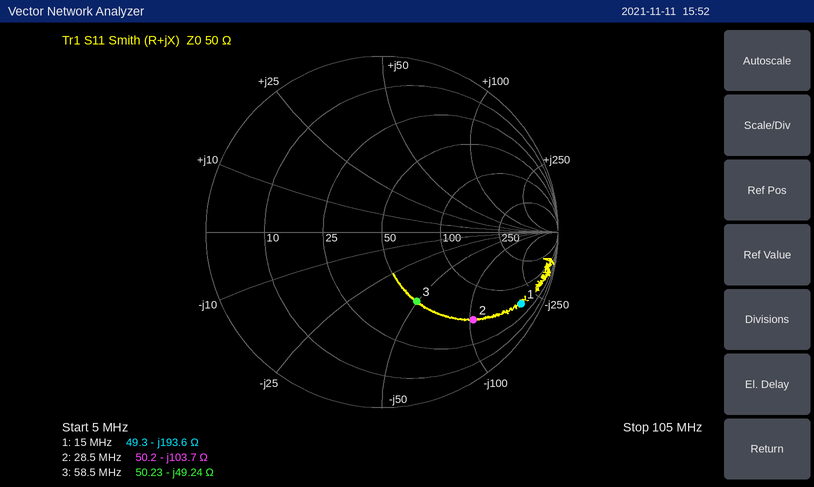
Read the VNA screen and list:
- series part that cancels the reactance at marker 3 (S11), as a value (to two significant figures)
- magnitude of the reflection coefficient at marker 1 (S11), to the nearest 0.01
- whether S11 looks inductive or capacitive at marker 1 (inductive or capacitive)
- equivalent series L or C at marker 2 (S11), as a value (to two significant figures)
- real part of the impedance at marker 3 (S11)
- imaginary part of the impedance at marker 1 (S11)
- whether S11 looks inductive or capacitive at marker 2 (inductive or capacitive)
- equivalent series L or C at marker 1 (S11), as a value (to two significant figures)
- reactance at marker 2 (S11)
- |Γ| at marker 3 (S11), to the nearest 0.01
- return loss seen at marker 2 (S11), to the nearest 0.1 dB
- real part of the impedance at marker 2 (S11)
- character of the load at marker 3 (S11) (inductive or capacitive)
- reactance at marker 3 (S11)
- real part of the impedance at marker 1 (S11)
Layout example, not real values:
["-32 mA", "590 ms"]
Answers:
["130 nH", "0.89", "capacitive", "54 pF", "50.23 Ω", "-193.6 Ω", "capacitive", "55 pF", "-103.7 Ω", "0.44", "2.9 dB", "50.2 Ω", "capacitive", "-49.24 Ω", "49.3 Ω"]
